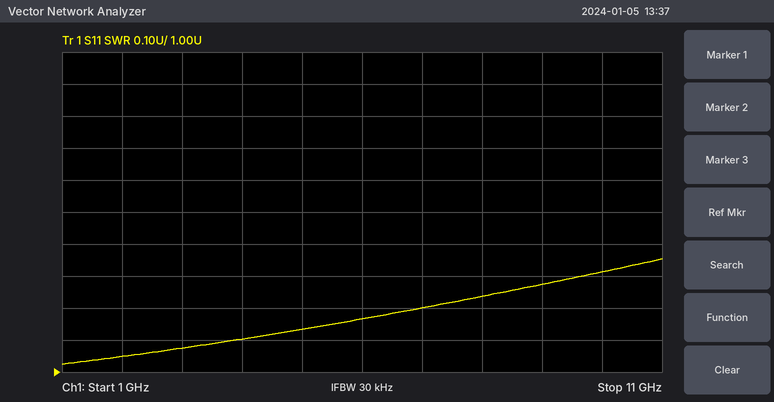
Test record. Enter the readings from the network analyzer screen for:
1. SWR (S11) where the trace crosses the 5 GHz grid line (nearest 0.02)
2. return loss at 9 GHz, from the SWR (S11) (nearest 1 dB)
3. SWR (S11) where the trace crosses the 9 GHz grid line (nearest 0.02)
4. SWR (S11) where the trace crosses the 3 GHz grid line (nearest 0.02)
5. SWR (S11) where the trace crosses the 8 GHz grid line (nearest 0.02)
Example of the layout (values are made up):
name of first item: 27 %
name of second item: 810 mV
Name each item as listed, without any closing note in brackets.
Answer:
SWR (S11) where the trace crosses the 5 GHz grid line: 1.14
return loss at 9 GHz, from the SWR (S11): 18 dB
SWR (S11) where the trace crosses the 9 GHz grid line: 1.28
SWR (S11) where the trace crosses the 3 GHz grid line: 1.08
SWR (S11) where the trace crosses the 8 GHz grid line: 1.24
